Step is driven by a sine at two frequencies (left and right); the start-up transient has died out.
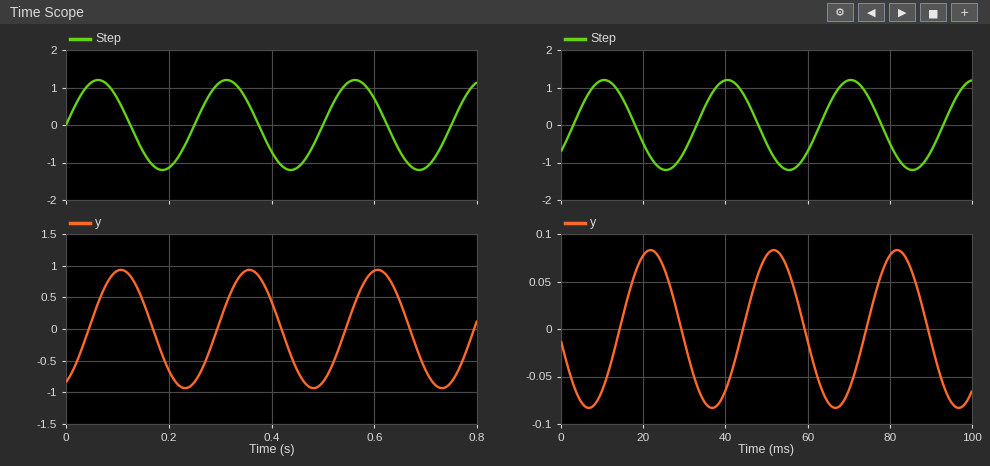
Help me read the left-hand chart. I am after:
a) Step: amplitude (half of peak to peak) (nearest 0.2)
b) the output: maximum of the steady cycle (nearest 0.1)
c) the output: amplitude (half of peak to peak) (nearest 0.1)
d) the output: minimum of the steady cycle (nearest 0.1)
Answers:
1.2
0.9
0.9
-0.9
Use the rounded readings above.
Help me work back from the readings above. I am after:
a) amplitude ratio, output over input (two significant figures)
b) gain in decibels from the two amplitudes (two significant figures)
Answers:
0.75
-2.5 dB
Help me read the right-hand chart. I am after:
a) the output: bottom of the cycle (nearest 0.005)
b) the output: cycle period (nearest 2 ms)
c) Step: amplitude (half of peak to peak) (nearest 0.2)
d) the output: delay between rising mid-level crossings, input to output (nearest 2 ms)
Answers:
-0.085
30 ms
1.2
12 ms
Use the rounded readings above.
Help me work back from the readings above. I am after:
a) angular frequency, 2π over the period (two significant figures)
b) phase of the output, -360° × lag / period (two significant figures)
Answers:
0.21 rad/ms
-140°
